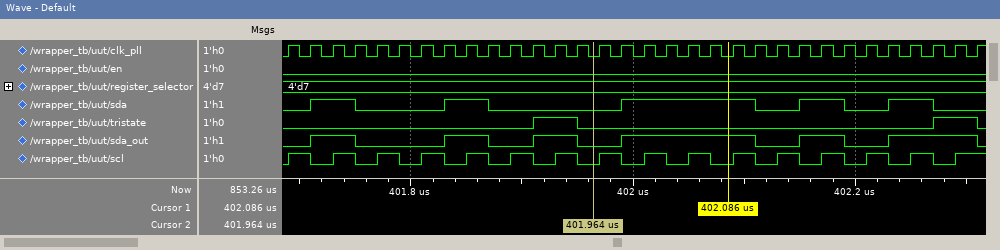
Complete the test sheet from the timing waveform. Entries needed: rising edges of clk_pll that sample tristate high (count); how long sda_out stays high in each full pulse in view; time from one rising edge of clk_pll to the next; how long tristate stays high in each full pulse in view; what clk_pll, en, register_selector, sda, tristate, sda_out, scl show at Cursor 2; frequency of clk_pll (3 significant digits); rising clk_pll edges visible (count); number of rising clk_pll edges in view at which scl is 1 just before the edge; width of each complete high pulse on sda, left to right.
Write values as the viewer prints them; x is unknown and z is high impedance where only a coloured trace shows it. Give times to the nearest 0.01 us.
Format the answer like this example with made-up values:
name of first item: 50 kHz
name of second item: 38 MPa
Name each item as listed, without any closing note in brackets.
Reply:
rising edges of clk_pll that sample tristate high: 4
how long sda_out stays high in each full pulse in view: 0.04 us, 0.04 us, 0.04 us, 0.12 us, 0.04 us, 0.08 us
time from one rising edge of clk_pll to the next: 0.02 us
how long tristate stays high in each full pulse in view: 0.04 us, 0.04 us
what clk_pll, en, register_selector, sda, tristate, sda_out, scl show at Cursor 2: clk_pll=0, en=0, register_selector=4'd7, sda=0, tristate=0, sda_out=0, scl=0
frequency of clk_pll: 50.0 MHz
rising clk_pll edges visible: 32
number of rising clk_pll edges in view at which scl is 1 just before the edge: 16
width of each complete high pulse on sda, left to right: 0.04 us, 0.04 us, 0.12 us, 0.04 us, 0.04 us
